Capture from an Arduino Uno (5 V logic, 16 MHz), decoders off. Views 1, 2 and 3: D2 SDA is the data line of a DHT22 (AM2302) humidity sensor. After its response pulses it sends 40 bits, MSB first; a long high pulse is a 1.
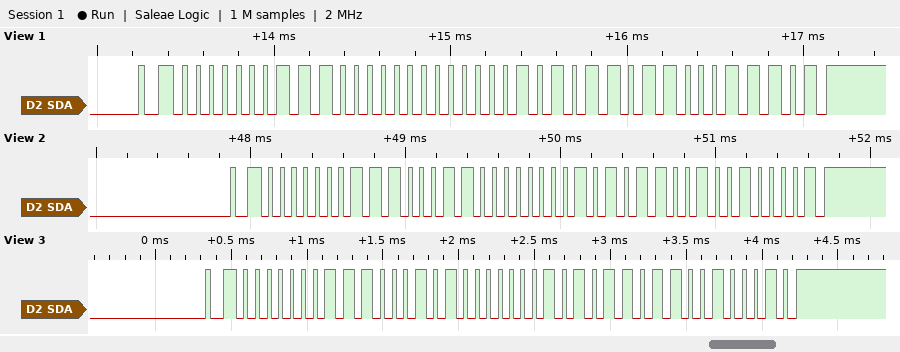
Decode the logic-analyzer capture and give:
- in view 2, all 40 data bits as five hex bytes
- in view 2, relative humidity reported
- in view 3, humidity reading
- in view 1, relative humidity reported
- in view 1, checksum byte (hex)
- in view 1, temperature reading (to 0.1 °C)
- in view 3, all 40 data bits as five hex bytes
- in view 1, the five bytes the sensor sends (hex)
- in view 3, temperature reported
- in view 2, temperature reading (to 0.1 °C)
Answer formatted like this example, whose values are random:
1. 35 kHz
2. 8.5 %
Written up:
1. 01 C6 01 59 21
2. 45.4 %
3. 45.3 %
4. 44.8 %
5. 0x1D
6. 34.7 °C
7. 01 C5 01 5B 22
8. 01 C0 01 5B 1D
9. 34.7 °C
10. 34.5 °C
